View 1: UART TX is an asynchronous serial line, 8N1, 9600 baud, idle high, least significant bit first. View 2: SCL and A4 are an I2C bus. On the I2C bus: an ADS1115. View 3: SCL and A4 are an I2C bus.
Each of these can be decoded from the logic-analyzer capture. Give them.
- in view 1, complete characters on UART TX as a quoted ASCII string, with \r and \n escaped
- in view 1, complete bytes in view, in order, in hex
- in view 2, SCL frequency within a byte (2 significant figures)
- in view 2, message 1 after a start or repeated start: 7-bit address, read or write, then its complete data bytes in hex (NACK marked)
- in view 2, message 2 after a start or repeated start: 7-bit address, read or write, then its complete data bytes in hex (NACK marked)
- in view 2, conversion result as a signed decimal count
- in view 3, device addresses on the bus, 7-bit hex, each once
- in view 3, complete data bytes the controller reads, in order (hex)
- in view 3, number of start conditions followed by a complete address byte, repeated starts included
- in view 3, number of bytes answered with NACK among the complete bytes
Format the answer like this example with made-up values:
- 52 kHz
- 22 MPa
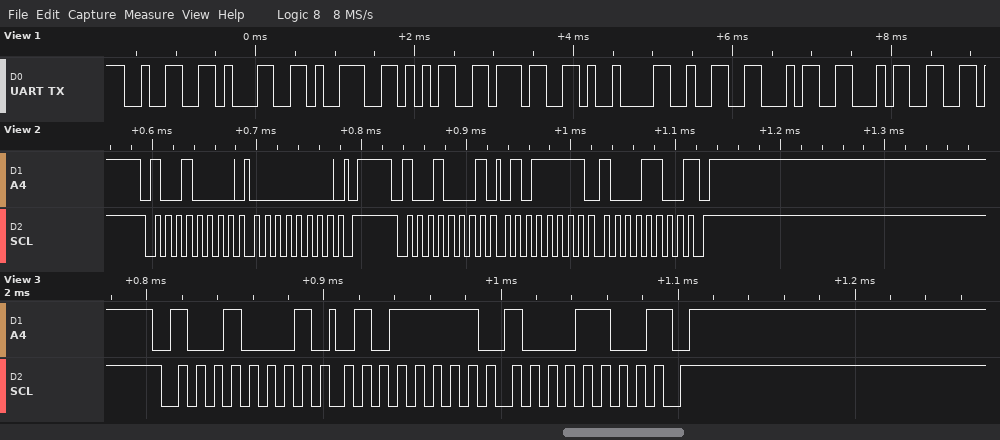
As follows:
- "21957\t244"
- 32 31 39 35 37 09 32 34 34
- 100 kHz
- 0x48 write: 00
- 0x48 read: 5F 8C NACK
- 24460
- 0x48
- 5F 8C
- 1
- 1
